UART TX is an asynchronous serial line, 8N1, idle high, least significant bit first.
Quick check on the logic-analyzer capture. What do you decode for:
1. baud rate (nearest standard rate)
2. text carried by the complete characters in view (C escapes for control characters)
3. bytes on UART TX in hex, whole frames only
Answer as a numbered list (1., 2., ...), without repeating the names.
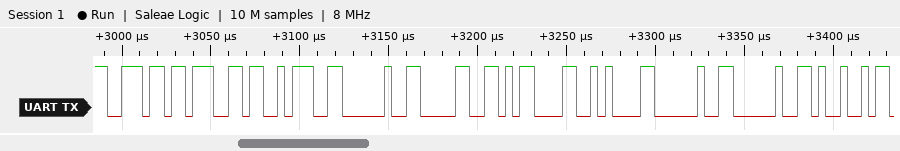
1. 250000 baud
2. "ng: 0\r\n  I"
3. 0x6E 0x67 0x3A 0x20 0x30 0x0D 0x0A 0x20 0x20 0x49
